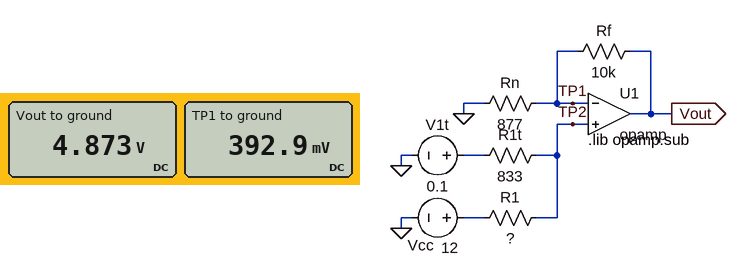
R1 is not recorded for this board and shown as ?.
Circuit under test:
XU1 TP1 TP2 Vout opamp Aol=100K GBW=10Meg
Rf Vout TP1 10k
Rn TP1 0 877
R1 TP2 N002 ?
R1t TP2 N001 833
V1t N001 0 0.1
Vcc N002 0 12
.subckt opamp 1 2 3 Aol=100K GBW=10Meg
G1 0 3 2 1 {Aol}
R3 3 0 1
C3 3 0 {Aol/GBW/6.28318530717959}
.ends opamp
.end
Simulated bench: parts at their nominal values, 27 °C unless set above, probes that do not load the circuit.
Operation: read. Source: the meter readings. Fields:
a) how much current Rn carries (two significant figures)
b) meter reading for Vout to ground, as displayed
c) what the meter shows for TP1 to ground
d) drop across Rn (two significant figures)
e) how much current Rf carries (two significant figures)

450 µA
4.873 V
392.9 mV
390 mV
450 µA
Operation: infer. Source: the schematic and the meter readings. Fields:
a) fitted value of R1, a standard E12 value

33 kΩ
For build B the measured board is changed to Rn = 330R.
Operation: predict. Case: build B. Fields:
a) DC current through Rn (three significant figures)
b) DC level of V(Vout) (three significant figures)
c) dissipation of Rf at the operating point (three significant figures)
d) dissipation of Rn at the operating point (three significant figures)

1.19 mA
12.3 V
14.2 mW
468 µW
